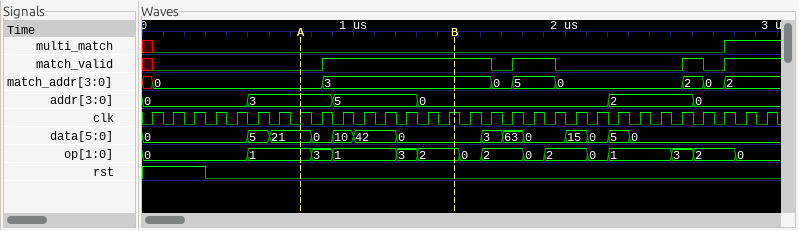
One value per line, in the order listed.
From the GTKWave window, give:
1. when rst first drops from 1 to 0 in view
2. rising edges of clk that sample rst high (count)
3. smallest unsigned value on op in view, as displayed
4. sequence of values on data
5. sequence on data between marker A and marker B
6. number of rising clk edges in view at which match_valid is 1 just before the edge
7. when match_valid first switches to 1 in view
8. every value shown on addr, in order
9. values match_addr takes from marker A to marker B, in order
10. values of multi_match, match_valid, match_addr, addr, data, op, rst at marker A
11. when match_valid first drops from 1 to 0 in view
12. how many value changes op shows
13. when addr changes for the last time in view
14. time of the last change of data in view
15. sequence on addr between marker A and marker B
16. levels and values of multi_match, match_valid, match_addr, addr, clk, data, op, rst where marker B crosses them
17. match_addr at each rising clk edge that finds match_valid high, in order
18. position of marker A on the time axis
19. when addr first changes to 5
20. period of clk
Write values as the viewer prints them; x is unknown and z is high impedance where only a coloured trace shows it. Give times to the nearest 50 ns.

300 ns
3
0
0, 5, 21, 0, 10, 42, 0, 3, 63, 0, 15, 0, 5, 0
21, 0, 10, 42, 0
13
850 ns
0, 3, 5, 0, 2, 0
0, 3
multi_match=0, match_valid=0, match_addr=0, addr=3, data=21, op=1, rst=0
1650 ns
14
2600 ns
2300 ns
3, 5, 0
multi_match=0, match_valid=1, match_addr=3, addr=0, clk=1, data=0, op=2, rst=0
3, 3, 3, 3, 3, 3, 3, 3, 5, 5, 2, 2, 2
750 ns
900 ns
100 ns
